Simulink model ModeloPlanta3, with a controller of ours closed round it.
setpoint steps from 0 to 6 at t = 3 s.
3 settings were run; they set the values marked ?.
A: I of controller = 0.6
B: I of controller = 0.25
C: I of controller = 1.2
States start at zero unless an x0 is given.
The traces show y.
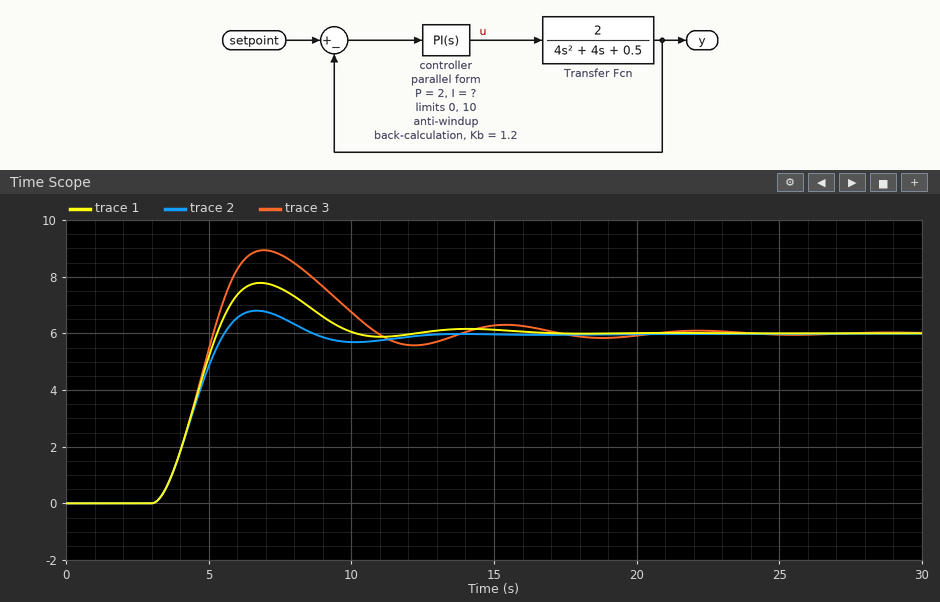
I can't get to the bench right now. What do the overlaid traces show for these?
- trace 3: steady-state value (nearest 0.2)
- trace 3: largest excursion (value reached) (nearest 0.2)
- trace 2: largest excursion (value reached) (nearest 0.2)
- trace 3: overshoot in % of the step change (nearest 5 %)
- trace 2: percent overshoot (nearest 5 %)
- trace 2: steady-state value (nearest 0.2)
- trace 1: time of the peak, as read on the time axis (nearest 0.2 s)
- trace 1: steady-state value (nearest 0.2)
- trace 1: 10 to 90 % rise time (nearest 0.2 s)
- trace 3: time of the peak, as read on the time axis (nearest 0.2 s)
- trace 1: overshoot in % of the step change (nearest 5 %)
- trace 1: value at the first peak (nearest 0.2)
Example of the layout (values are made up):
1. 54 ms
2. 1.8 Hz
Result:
1. 6.0
2. 9.0
3. 6.8
4. 50 %
5. 15 %
6. 6.0
7. 6.8 s
8. 6.0
9. 1.6 s
10. 7.0 s
11. 30 %
12. 7.8
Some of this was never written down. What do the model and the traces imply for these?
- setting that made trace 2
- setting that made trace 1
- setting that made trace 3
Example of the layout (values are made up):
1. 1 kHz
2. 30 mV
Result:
1. B
2. A
3. C
